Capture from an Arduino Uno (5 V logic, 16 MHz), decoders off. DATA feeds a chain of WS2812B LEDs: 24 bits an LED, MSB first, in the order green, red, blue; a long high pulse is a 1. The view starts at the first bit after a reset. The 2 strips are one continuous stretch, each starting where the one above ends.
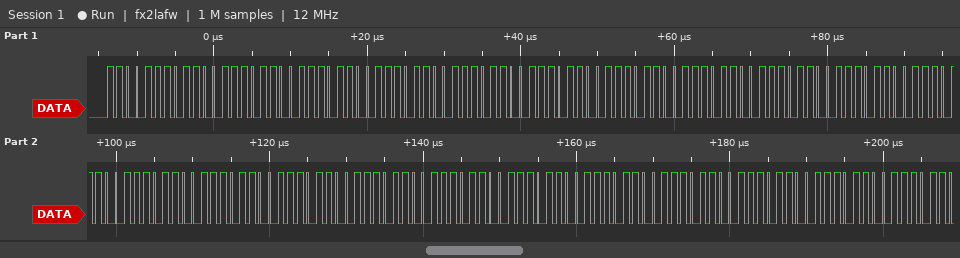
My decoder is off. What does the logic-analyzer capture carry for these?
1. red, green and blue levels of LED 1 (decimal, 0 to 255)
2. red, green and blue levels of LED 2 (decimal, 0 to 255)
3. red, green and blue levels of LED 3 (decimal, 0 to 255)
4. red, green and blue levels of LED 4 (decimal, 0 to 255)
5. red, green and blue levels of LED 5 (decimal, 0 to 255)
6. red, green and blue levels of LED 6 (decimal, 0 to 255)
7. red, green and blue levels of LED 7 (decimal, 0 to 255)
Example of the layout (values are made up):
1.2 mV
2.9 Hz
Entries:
206, 206, 206
206, 206, 206
206, 206, 206
206, 206, 206
206, 206, 206
206, 206, 206
206, 206, 206
